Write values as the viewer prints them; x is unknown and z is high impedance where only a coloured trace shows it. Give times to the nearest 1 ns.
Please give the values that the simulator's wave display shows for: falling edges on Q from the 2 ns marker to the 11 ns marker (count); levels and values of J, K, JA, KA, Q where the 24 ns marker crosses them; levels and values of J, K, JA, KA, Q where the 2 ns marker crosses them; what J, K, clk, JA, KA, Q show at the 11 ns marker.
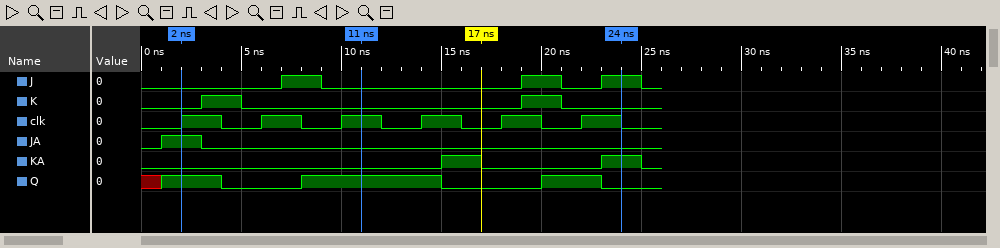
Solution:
1
J=1, K=0, JA=0, KA=1, Q=0
J=0, K=0, JA=1, KA=0, Q=1
J=0, K=0, clk=1, JA=0, KA=0, Q=1
